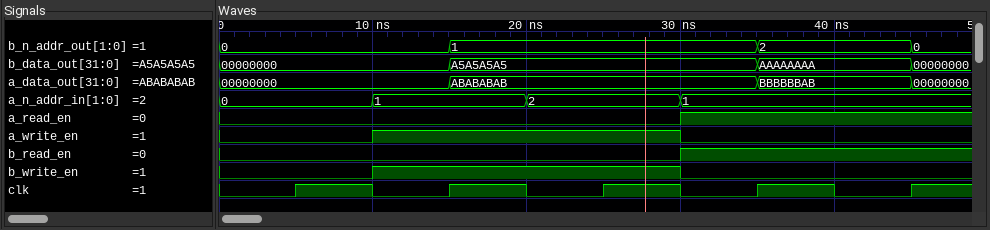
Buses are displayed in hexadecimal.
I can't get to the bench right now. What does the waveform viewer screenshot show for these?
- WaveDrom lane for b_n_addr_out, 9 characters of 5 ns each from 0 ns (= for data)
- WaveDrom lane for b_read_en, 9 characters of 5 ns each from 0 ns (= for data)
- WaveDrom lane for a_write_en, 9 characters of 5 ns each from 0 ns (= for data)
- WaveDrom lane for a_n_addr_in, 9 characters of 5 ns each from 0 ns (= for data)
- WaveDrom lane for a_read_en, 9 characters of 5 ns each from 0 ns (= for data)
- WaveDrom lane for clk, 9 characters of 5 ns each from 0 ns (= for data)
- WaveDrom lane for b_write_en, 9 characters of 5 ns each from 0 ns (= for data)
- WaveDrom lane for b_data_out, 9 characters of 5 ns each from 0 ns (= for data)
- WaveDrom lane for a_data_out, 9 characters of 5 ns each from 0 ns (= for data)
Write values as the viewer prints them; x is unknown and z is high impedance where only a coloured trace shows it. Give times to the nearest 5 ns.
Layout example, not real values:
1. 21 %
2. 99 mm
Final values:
1. {name: 'b_n_addr_out', wave: '=..=...=.', data: '0 1 2'}
2. {name: 'b_read_en', wave: '0.....1..'}
3. {name: 'a_write_en', wave: '0.1...0..'}
4. {name: 'a_n_addr_in', wave: '=.=.=.=..', data: '0 1 2 1'}
5. {name: 'a_read_en', wave: '0.....1..'}
6. {name: 'clk', wave: '010101010'}
7. {name: 'b_write_en', wave: '0.1...0..'}
8. {name: 'b_data_out', wave: '=..=...=.', data: '00000000 A5A5A5A5 AAAAAAAA'}
9. {name: 'a_data_out', wave: '=..=...=.', data: '00000000 ABABABAB BBBBBBAB'}
